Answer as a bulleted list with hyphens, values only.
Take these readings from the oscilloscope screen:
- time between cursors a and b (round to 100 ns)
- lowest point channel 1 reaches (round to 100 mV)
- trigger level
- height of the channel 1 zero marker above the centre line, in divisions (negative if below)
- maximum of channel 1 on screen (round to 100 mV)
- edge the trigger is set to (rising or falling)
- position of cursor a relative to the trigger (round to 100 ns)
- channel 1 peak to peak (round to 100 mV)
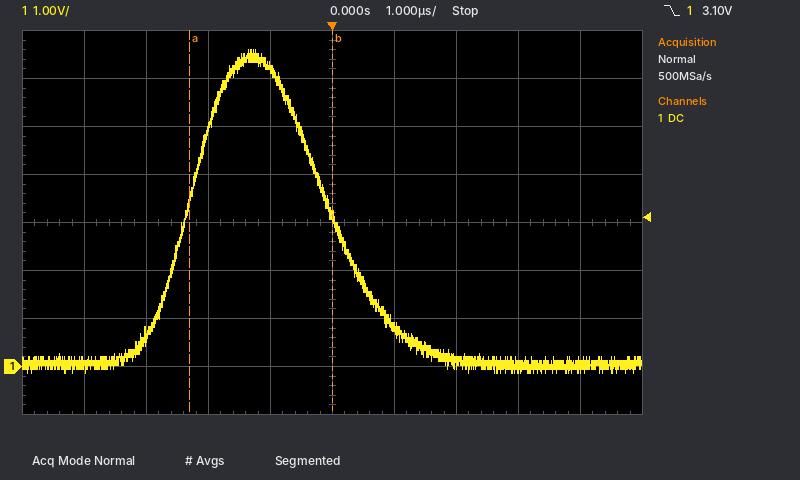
- 2.3 µs
- -100 mV
- 3.10 V
- -3.0 div
- 6.6 V
- falling
- -2.3 µs
- 6.7 V
